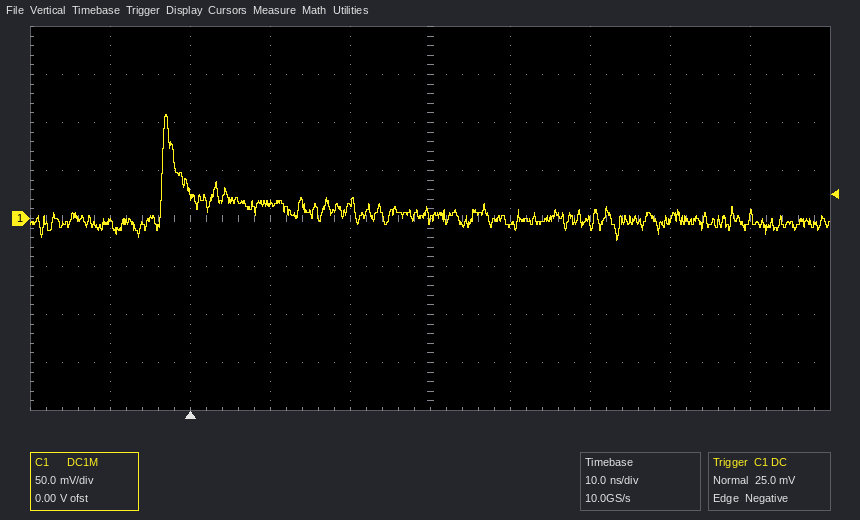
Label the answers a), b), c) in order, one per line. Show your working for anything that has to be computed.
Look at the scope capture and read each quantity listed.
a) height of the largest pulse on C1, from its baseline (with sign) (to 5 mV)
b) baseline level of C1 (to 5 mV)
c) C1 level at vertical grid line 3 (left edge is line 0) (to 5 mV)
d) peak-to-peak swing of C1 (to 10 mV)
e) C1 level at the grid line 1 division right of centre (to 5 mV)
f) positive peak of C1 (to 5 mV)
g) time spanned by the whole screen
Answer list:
a) 110 mV − (0 mV) = +110 mV
b) 0 mV
c) 15 mV
d) 130 mV
e) -5 mV
f) 110 mV
g) 100 ns
